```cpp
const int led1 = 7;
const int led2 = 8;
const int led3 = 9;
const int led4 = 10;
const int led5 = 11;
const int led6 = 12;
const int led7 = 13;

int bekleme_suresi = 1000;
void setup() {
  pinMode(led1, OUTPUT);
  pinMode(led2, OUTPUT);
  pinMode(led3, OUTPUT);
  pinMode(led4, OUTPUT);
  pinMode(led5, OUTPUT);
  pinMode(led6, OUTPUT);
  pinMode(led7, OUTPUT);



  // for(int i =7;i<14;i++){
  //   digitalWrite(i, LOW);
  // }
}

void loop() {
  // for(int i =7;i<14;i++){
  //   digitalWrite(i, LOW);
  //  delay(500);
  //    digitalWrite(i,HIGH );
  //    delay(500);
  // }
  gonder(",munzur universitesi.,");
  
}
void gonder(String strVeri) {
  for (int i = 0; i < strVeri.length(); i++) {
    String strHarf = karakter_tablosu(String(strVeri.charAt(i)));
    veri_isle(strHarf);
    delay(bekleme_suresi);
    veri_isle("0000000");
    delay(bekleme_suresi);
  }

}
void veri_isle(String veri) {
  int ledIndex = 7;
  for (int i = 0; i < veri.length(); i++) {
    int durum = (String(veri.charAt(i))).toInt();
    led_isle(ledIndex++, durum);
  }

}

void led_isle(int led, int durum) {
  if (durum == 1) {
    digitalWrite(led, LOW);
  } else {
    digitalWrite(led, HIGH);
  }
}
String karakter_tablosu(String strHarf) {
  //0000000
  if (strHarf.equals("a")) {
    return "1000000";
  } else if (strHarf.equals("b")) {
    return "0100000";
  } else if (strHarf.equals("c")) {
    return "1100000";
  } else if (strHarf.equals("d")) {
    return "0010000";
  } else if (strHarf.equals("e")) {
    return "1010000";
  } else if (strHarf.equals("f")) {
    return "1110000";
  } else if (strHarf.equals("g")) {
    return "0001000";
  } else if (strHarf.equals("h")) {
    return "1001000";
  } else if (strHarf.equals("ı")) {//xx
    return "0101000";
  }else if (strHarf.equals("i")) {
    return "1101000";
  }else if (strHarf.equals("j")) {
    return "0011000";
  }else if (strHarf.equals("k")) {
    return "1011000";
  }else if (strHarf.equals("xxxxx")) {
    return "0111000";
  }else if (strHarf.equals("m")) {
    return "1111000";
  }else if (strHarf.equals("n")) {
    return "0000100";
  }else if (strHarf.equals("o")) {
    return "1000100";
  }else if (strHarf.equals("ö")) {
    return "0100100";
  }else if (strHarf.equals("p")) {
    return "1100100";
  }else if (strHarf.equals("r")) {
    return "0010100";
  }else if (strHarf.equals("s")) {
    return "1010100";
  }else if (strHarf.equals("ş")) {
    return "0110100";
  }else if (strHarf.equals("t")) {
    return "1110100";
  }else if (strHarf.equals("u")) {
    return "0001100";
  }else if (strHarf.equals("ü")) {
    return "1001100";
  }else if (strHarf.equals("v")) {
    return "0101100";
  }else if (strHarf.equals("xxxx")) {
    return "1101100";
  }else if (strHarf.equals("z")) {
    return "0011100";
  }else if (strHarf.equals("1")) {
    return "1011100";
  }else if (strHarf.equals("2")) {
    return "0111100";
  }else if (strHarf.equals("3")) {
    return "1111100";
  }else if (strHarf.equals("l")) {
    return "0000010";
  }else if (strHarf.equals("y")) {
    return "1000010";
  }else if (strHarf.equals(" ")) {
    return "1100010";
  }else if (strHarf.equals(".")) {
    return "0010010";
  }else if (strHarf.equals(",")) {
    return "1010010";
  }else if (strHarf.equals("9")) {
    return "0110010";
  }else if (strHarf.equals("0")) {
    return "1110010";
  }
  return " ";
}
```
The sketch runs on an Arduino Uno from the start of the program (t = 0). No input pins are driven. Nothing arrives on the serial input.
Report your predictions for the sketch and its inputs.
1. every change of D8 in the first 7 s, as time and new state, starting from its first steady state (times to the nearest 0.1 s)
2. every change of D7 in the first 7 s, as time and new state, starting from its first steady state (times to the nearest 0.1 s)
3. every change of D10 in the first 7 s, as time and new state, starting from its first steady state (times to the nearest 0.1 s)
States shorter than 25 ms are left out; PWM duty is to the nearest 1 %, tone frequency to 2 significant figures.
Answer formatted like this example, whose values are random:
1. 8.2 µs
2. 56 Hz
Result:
1. 0 s high; 2 s low; 3 s high
2. 0 s low; 1 s high; 2 s low; 3 s high
3. 0 s high; 2 s low; 3 s high; 4 s low; 5 s high
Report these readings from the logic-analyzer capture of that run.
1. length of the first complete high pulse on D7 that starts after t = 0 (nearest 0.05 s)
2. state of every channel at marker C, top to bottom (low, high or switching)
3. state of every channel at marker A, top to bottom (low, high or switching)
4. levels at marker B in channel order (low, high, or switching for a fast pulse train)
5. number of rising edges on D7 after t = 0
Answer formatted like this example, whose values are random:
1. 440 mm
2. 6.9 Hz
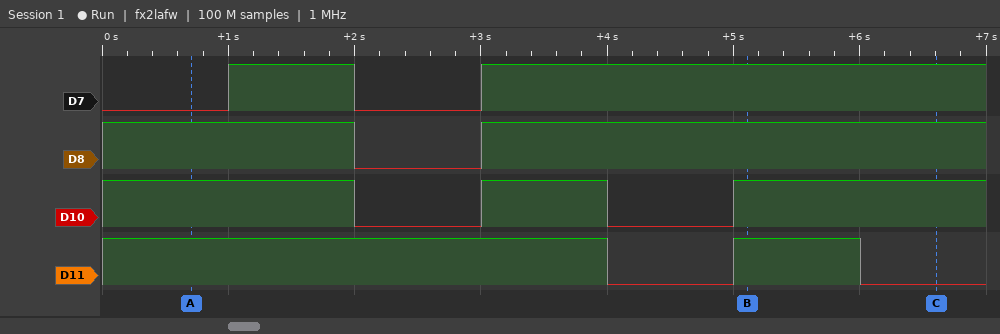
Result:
1. 1.00 s
2. D7 high, D8 high, D10 high, D11 low
3. D7 low, D8 high, D10 high, D11 high
4. D7 high, D8 high, D10 high, D11 high
5. 2
